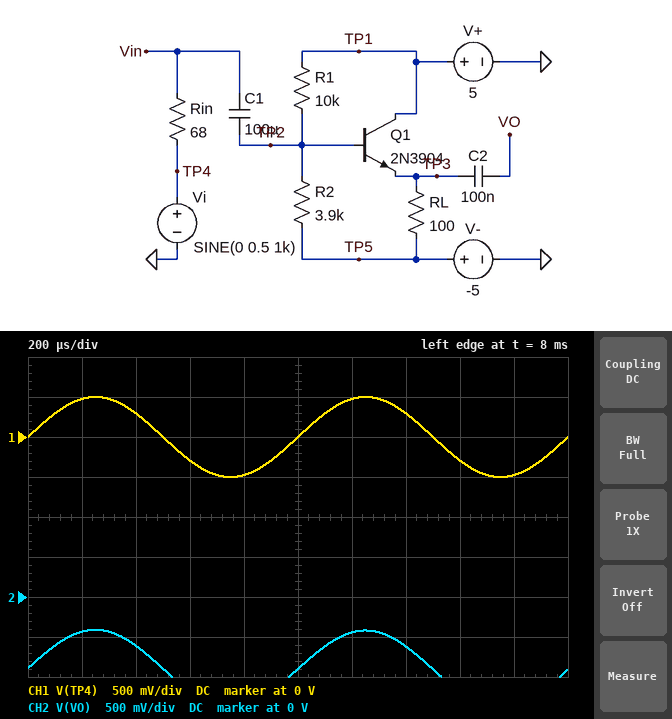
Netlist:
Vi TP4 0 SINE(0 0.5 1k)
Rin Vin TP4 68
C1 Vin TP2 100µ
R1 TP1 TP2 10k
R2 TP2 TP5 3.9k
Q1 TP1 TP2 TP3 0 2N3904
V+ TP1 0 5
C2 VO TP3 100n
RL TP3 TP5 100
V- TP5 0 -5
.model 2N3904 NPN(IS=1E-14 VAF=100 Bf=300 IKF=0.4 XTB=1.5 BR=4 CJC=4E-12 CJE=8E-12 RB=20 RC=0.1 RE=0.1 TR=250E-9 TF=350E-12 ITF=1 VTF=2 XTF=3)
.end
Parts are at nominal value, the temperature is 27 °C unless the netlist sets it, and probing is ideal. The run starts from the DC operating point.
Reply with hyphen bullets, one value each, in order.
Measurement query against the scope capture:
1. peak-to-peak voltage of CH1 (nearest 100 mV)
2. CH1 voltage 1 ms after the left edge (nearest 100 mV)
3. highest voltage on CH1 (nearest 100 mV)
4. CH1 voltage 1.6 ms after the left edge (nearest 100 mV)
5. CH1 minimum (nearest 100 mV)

- 1.0 V
- 0 V
- 500 mV
- -300 mV
- -500 mV
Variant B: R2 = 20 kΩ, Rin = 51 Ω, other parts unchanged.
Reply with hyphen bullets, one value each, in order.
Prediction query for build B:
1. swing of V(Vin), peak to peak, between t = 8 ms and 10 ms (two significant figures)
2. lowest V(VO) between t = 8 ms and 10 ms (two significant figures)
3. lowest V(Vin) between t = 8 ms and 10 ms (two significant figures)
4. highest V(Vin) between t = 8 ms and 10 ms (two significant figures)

- 990 mV
- -1.2 V
- -490 mV
- 500 mV
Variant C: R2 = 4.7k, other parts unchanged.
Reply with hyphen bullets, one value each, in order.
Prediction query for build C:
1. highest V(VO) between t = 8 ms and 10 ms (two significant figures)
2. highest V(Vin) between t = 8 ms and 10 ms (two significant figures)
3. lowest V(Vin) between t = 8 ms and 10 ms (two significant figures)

- -380 mV
- 440 mV
- -530 mV
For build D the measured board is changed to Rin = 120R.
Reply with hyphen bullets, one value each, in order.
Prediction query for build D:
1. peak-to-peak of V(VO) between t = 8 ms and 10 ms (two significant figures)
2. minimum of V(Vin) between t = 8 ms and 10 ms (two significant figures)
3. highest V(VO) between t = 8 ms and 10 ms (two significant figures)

- 960 mV
- -580 mV
- -460 mV
